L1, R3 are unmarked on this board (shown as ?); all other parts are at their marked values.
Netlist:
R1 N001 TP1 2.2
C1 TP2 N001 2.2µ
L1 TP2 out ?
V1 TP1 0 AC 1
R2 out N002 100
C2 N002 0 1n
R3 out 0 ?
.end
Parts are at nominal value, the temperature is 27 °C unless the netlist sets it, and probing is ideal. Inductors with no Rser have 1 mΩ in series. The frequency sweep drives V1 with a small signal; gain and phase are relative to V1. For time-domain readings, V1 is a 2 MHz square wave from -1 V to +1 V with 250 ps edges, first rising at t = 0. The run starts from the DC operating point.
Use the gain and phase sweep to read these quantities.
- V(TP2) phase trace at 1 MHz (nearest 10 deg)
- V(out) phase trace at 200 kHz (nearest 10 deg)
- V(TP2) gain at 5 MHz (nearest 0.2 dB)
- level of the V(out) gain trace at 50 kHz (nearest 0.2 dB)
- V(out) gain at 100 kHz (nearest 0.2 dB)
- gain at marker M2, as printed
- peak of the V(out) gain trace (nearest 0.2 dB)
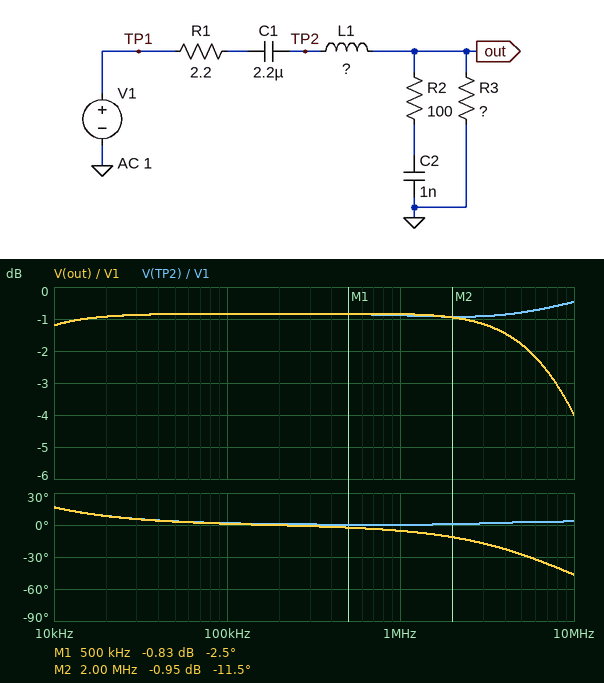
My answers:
0 deg
0 deg
-0.8 dB
-0.8 dB
-0.8 dB
-0.95 dB
-0.8 dB
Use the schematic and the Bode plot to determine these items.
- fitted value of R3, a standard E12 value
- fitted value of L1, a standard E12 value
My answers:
22 Ω
330 nH
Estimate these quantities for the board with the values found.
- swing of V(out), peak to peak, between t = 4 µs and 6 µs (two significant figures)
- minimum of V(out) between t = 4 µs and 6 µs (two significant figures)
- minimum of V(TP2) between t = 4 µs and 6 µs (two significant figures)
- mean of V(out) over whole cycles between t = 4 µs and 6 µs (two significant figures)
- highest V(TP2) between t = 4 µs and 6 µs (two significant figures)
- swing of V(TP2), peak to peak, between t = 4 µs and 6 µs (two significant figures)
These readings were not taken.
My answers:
1.9 V
-100 mV
-280 mV
830 mV
1.9 V
2.2 V
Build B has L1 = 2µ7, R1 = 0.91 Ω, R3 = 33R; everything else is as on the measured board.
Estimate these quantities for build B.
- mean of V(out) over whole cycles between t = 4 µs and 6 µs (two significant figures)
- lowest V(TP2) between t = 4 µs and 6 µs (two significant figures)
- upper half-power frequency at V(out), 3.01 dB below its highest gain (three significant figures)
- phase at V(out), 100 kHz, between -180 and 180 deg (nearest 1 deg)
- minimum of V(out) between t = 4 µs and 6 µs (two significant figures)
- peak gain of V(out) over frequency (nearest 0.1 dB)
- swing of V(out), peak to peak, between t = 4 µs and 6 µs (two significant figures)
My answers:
910 mV
-130 mV
1.89 MHz
-2 deg
-6.3 mV
-0.2 dB
1.8 V
